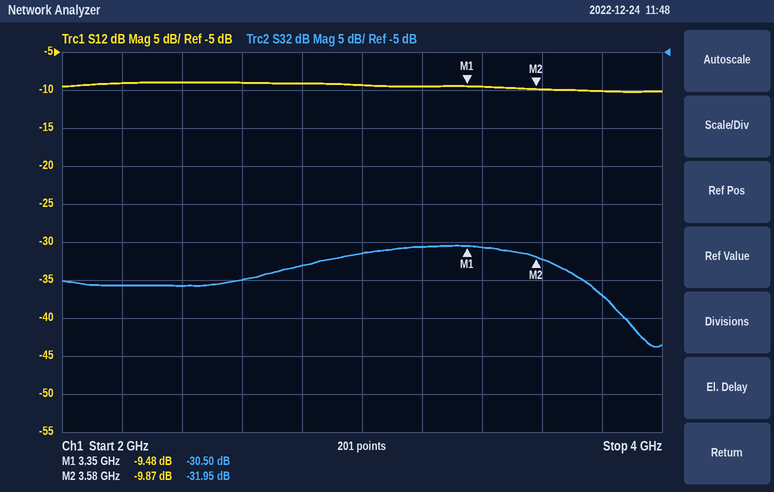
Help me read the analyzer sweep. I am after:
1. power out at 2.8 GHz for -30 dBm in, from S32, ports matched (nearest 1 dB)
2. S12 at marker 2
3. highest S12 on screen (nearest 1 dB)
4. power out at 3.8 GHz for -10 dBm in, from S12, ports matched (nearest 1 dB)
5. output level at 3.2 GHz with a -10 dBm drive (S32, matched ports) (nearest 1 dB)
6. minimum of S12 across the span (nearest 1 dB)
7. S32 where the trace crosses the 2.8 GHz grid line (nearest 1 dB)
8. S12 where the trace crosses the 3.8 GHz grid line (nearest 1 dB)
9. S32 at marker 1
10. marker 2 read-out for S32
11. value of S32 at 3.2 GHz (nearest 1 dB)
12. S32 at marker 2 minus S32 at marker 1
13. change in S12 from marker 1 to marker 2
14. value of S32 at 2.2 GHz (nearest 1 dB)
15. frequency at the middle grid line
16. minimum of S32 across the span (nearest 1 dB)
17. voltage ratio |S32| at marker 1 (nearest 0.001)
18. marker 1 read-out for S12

-63 dBm
-9.87 dB
-9 dB
-20 dBm
-41 dBm
-10 dB
-33 dB
-10 dB
-30.50 dB
-31.95 dB
-31 dB
-1.45 dB
-0.39 dB
-36 dB
3 GHz
-44 dB
0.030
-9.48 dB
